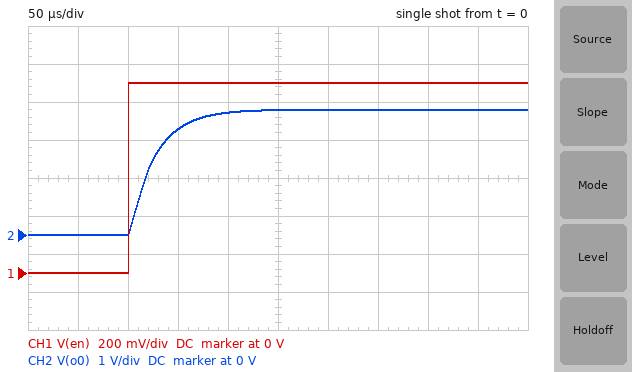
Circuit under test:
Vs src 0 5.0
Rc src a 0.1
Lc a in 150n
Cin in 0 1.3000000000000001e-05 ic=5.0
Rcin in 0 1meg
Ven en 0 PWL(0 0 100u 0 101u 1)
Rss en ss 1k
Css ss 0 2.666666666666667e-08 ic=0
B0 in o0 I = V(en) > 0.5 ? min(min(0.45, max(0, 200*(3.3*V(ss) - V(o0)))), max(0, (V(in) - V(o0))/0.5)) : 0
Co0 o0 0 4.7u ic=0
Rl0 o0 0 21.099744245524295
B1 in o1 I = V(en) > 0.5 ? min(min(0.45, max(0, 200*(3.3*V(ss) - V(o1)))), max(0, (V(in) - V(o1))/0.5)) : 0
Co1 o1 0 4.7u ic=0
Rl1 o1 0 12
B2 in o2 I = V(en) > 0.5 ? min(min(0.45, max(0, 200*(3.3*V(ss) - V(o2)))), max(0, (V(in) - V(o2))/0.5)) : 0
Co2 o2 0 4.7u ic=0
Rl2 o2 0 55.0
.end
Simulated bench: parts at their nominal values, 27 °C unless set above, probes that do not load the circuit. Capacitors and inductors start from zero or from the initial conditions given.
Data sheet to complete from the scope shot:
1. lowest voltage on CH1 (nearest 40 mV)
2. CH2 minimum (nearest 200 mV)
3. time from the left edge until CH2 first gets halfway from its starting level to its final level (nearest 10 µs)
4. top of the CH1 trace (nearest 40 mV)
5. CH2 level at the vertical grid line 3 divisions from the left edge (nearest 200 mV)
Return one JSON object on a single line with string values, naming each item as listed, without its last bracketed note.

{"lowest voltage on CH1": "0 V", "CH2 minimum": "0 V", "time from the left edge until CH2 first gets halfway from its starting level to its final level": "120 µs", "top of the CH1 trace": "1.00 V", "CH2 level at the vertical grid line 3 divisions from the left edge": "2.8 V"}
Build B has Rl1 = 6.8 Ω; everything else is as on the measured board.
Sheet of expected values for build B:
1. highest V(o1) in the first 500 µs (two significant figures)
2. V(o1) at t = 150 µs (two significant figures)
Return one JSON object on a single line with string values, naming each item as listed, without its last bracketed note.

{"highest V(o1) in the first 500 µs": "3.1 V", "V(o1) at t = 150 µs": "2.4 V"}
